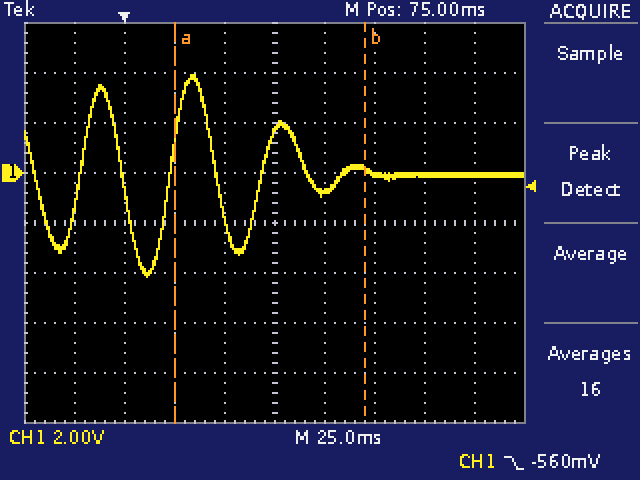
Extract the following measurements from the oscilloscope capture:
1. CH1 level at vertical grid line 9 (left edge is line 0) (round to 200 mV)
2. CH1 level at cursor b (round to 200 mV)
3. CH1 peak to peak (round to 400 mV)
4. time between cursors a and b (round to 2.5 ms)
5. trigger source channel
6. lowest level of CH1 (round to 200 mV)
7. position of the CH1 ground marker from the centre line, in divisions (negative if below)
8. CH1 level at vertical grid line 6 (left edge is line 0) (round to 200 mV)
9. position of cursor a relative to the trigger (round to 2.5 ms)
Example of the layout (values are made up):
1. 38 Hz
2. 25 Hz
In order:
1. 0.0 V
2. 200 mV
3. 8.0 V
4. 95.0 ms
5. CH1
6. -4.2 V
7. +1.0 div
8. -800 mV
9. +25.0 ms
